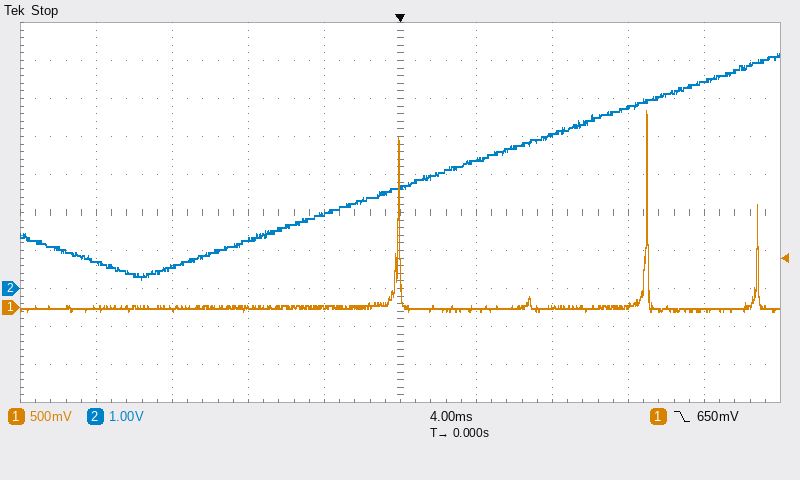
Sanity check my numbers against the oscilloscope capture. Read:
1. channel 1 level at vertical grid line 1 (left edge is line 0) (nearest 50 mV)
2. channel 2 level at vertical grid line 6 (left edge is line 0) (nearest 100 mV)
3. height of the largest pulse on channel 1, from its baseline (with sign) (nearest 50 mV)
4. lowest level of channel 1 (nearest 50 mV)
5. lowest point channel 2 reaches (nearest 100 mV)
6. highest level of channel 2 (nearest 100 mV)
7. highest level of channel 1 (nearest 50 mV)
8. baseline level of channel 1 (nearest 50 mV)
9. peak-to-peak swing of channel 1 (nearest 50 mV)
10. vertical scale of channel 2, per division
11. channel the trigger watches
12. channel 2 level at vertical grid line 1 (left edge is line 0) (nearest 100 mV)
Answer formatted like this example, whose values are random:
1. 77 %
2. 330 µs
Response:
1. 0 mV
2. 3.4 V
3. +2.60 V
4. -50 mV
5. 200 mV
6. 6.2 V
7. 2.60 V
8. 0 mV
9. 2.65 V
10. 1 V
11. channel 1
12. 700 mV
